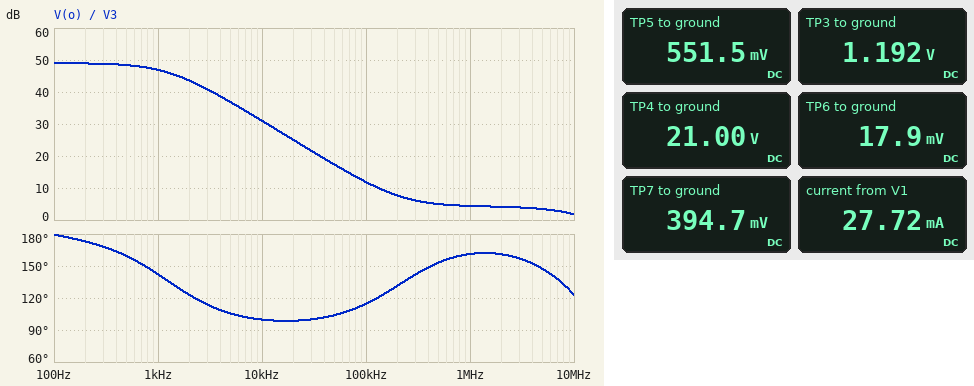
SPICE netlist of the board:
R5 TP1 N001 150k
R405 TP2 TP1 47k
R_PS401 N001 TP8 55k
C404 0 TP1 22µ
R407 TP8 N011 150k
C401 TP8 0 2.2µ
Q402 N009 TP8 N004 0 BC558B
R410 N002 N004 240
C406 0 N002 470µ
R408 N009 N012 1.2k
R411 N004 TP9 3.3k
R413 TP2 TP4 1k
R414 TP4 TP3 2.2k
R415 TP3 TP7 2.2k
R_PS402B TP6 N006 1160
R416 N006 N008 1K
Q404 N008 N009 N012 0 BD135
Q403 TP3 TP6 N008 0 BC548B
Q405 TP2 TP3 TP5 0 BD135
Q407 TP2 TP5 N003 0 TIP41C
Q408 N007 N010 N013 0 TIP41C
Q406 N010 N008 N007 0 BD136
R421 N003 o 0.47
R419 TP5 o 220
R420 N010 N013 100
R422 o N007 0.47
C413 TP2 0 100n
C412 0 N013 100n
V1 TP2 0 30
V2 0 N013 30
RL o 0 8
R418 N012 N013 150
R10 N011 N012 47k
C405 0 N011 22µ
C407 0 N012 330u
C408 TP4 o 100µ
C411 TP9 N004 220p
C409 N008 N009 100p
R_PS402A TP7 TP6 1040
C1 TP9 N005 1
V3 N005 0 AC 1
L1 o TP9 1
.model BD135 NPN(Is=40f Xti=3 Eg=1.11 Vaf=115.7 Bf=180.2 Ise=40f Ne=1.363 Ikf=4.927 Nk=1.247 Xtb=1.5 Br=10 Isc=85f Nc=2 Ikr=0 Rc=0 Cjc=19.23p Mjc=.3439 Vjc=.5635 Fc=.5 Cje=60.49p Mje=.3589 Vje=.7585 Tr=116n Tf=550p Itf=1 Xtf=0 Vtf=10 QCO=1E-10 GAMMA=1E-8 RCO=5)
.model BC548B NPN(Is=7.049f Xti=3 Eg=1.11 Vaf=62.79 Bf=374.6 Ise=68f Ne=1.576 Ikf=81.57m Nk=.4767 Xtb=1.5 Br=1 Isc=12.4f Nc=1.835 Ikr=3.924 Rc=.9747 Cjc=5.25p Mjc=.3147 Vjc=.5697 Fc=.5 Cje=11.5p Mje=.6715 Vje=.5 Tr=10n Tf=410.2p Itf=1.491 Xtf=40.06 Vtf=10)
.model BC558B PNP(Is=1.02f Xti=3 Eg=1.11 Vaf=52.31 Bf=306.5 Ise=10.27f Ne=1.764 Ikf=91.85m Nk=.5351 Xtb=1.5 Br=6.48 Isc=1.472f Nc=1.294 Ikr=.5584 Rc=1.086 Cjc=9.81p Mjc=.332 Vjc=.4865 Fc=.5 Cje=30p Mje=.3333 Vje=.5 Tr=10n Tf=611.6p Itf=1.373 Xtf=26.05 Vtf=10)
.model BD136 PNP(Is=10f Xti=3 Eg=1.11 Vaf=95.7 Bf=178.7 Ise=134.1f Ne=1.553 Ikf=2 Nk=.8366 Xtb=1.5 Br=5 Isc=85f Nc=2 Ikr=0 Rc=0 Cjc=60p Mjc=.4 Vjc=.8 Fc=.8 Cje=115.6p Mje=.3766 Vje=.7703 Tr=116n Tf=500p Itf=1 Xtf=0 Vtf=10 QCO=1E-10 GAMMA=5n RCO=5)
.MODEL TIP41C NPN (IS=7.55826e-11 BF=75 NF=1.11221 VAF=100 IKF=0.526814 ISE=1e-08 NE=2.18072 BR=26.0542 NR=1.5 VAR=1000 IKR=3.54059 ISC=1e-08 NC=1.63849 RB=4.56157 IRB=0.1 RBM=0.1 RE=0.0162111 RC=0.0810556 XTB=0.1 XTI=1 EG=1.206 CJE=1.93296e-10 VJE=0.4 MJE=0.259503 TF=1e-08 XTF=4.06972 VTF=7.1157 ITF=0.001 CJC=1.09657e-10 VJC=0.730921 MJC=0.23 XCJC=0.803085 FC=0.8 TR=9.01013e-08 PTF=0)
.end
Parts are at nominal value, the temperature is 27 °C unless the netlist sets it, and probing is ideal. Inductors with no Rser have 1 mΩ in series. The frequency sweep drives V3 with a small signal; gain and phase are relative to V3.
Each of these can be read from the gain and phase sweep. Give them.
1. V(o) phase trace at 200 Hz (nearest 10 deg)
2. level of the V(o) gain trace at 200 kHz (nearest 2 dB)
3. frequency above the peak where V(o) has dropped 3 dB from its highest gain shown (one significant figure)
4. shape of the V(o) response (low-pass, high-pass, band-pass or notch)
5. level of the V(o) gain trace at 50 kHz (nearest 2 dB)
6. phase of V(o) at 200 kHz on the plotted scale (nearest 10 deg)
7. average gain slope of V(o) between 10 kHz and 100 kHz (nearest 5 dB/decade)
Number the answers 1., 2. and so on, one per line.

1. 170 deg
2. 8 dB
3. 1 kHz
4. low-pass
5. 18 dB
6. 130 deg
7. -20 dB/decade
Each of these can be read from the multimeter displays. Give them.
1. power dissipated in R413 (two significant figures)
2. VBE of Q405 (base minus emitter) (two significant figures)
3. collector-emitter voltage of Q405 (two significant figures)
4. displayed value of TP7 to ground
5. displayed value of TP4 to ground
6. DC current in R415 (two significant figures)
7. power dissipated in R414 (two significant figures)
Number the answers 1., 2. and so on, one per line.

1. 81 mW
2. 640 mV
3. 29 V
4. 394.7 mV
5. 21.00 V
6. 360 µA
7. 180 mW
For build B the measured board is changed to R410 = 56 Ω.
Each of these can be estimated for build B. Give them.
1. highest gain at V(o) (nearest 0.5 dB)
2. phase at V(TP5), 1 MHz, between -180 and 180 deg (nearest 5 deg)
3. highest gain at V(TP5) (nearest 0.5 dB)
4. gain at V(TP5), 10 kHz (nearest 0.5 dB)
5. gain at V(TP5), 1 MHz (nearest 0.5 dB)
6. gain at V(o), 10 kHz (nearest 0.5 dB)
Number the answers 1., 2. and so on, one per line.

1. 45.5 dB
2. 165 deg
3. 46.0 dB
4. 28.0 dB
5. 1.5 dB
6. 27.5 dB
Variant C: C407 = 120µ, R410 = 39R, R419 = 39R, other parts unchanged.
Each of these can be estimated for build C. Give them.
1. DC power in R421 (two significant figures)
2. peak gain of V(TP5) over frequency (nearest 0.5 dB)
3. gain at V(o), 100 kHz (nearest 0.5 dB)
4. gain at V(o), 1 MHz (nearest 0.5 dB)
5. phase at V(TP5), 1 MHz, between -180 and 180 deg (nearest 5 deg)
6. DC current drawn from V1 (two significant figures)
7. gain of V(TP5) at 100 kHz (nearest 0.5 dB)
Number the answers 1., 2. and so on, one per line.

1. 11 µW
2. 44.0 dB
3. 7.0 dB
4. -0.5 dB
5. 165 deg
6. 27 mA
7. 7.5 dB
